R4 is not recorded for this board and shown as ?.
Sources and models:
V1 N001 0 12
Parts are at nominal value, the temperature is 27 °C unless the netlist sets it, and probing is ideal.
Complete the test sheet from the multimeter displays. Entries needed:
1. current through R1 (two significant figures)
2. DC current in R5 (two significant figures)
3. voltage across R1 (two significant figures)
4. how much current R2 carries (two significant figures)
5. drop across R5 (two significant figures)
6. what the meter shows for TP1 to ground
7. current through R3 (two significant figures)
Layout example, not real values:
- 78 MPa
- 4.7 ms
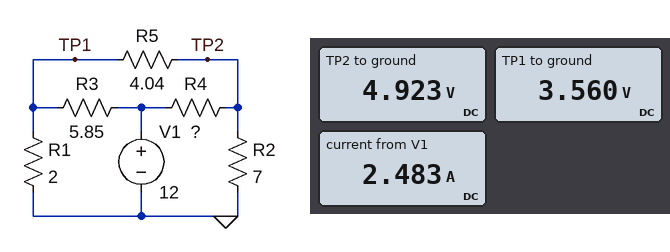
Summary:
- 1.8 A
- 340 mA
- 3.6 V
- 700 mA
- 1.4 V
- 3.560 V
- 1.4 A
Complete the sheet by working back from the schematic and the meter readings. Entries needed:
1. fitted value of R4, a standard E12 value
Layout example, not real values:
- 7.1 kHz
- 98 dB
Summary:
- 6.8 Ω
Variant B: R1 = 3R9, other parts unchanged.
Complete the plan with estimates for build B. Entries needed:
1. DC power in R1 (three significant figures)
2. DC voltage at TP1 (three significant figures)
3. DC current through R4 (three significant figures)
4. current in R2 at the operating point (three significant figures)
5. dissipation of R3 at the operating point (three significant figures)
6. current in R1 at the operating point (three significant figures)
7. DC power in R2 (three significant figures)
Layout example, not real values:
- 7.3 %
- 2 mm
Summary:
- 6.69 W
- 5.11 V
- 936 mA
- 805 mA
- 8.12 W
- 1.31 A
- 4.54 W
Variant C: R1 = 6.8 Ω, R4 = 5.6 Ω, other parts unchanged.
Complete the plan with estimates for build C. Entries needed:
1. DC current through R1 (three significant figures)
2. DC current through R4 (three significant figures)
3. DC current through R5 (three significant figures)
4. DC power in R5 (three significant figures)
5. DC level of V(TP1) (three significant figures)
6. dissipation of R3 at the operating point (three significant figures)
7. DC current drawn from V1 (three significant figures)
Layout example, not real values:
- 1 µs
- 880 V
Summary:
- 958 mA
- 964 mA
- 21.0 mA
- 1.78 mW
- 6.52 V
- 5.14 W
- 1.90 A
